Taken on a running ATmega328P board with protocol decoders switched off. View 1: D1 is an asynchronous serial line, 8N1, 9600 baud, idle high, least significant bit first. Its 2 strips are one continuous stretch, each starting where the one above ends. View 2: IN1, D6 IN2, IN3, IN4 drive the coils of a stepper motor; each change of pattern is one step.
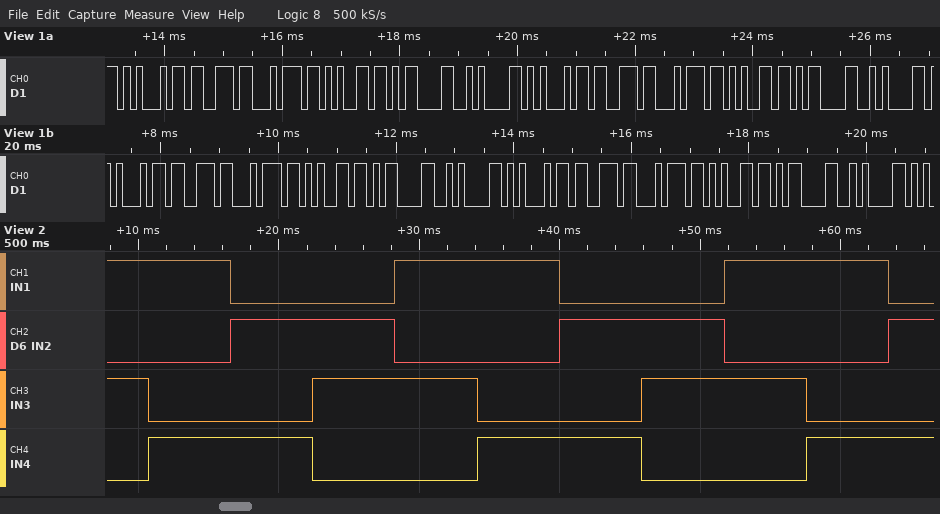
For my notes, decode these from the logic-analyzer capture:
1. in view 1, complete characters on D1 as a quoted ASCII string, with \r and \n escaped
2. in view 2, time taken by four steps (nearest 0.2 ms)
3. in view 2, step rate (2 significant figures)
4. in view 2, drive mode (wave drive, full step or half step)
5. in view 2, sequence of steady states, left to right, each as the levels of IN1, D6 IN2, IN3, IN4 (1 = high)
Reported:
"Este\r\nEste\r\nEste\r\nEste\r\n"
23.4 ms
170 steps/s
full step
1010 1001 0101 0110 1010 1001 0101 0110 1010 1001 0101
